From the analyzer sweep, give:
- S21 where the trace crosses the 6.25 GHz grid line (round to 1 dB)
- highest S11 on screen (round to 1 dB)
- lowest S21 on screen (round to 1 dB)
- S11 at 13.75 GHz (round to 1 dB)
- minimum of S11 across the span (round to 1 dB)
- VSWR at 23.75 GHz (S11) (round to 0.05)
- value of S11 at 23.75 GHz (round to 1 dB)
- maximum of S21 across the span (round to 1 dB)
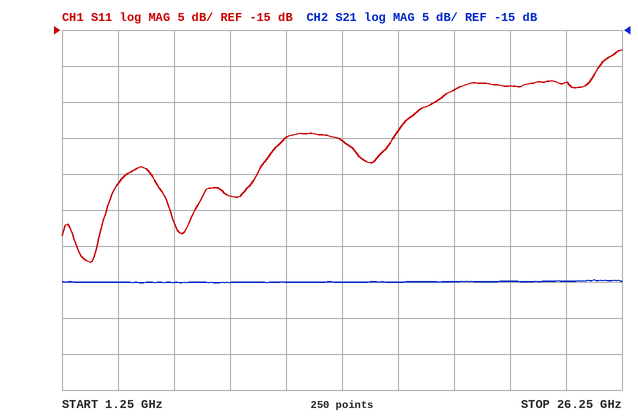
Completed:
-50 dB
-18 dB
-50 dB
-30 dB
-47 dB
1.15
-22 dB
-50 dB
